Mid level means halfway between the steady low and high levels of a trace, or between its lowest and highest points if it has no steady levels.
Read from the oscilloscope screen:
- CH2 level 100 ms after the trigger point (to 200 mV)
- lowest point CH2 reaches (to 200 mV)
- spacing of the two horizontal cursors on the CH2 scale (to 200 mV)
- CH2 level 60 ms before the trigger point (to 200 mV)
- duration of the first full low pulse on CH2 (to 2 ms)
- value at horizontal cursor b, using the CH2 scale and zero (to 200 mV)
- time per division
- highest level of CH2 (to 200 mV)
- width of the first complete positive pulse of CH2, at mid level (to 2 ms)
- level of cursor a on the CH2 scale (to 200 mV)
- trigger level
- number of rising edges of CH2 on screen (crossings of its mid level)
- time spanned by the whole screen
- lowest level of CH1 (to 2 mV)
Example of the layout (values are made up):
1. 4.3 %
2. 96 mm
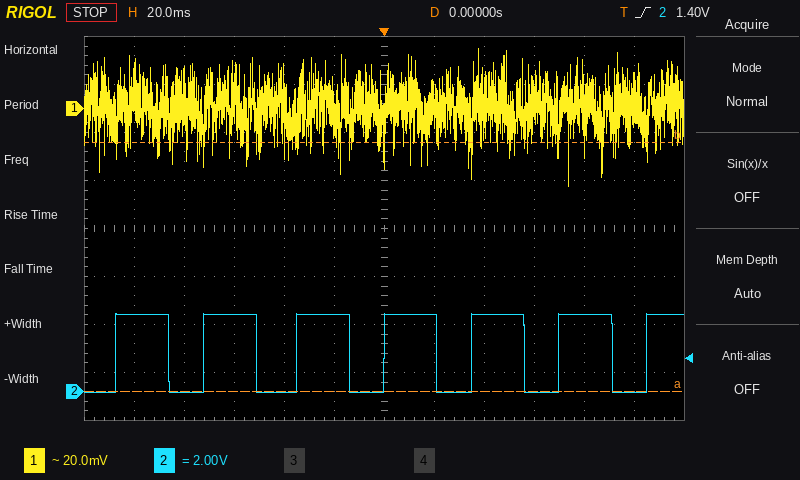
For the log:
1. 0.0 V
2. 0.0 V
3. 10.4 V
4. 3.2 V
5. 14 ms
6. 10.4 V
7. 20 ms
8. 3.2 V
9. 22 ms
10. 0.0 V
11. 1.40 V
12. 7
13. 240 ms
14. -32 mV
